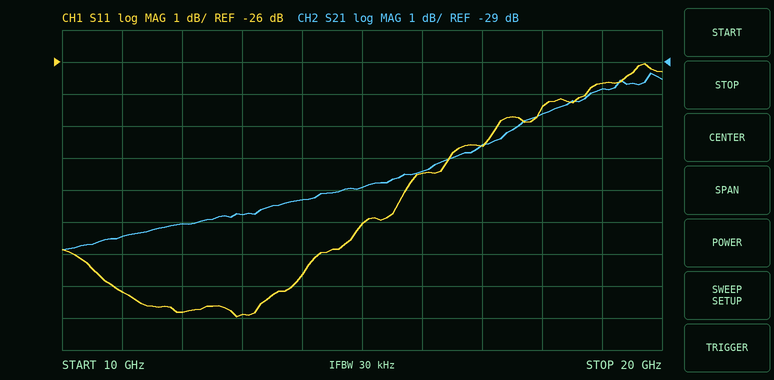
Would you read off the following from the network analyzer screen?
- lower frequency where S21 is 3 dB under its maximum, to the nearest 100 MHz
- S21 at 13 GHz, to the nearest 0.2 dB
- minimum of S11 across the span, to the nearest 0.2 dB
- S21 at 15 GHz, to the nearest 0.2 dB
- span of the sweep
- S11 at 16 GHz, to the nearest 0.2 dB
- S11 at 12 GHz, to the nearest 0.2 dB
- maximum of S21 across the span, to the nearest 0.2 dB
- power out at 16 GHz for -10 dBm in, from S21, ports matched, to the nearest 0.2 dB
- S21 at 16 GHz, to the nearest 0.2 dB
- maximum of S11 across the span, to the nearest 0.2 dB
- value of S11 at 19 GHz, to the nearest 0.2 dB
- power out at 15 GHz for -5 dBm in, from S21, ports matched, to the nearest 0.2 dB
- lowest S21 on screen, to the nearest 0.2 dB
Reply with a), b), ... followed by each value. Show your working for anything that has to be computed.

a) 16.1 GHz
b) -33.8 dB
c) -34.0 dB
d) -33.0 dB
e) 10 GHz
f) -29.4 dB
g) -33.8 dB
h) -29.4 dB
i) -10 dBm + (-32.4 dB) = -42.4 dBm
j) -32.4 dB
k) -26.0 dB
l) -26.6 dB
m) -5 dBm + (-33.0 dB) = -38.0 dBm
n) -34.8 dB
